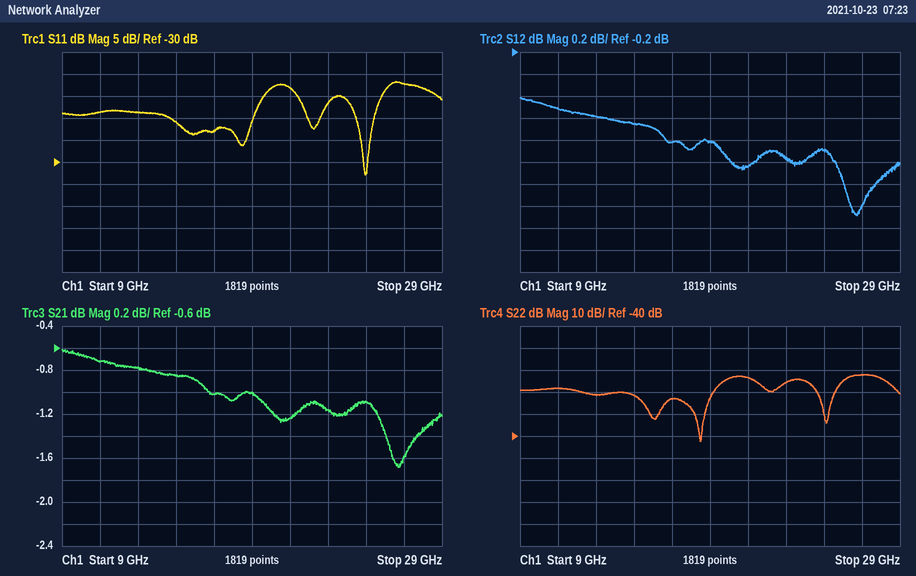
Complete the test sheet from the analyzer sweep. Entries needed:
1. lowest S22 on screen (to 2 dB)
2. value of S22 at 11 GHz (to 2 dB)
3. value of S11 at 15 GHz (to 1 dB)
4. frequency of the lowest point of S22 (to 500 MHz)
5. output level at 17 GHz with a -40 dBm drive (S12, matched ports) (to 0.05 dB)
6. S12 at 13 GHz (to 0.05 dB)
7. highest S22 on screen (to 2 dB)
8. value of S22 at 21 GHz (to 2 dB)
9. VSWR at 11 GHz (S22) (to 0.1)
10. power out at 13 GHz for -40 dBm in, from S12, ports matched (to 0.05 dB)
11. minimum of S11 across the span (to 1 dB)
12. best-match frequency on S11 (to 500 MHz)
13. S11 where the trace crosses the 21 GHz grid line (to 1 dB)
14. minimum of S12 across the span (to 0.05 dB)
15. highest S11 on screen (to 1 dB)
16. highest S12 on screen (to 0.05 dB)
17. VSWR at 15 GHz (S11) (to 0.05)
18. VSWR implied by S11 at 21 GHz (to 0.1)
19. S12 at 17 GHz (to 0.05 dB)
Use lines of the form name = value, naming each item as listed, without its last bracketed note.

lowest S22 on screen = -42 dB
value of S22 at 11 GHz = -18 dB
value of S11 at 15 GHz = -21 dB
frequency of the lowest point of S22 = 18.5 GHz
output level at 17 GHz with a -40 dBm drive (S12, matched ports) = -41.00 dBm
S12 at 13 GHz = -0.80 dB
highest S22 on screen = -12 dB
value of S22 at 21 GHz = -14 dB
VSWR at 11 GHz (S22) = 1.3
power out at 13 GHz for -40 dBm in, from S12, ports matched = -40.80 dBm
minimum of S11 across the span = -33 dB
best-match frequency on S11 = 25.0 GHz
S11 where the trace crosses the 21 GHz grid line = -13 dB
minimum of S12 across the span = -1.70 dB
highest S11 on screen = -12 dB
highest S12 on screen = -0.60 dB
VSWR at 15 GHz (S11) = 1.20
VSWR implied by S11 at 21 GHz = 1.6
S12 at 17 GHz = -1.00 dB
